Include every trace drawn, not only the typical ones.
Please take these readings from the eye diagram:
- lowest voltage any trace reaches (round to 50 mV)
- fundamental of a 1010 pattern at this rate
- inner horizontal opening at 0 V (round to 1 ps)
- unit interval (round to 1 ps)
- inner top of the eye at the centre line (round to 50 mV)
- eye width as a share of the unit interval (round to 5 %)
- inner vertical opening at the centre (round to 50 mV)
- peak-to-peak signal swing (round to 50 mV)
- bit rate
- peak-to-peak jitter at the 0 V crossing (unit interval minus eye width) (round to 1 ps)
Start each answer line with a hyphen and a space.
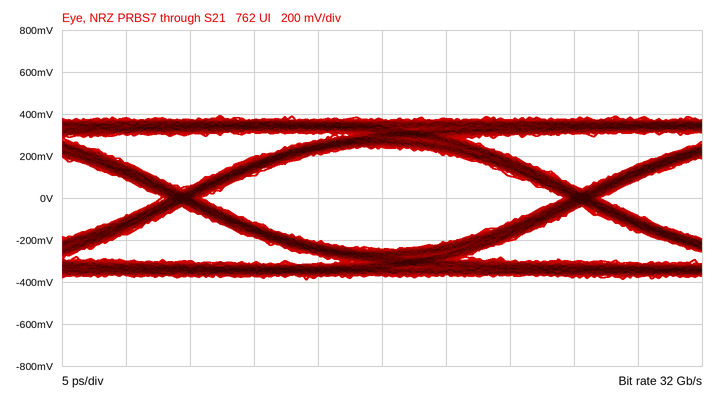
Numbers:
- -400 mV
- 16 GHz
- 28 ps
- 31 ps
- 250 mV
- 90 %
- 500 mV
- 800 mV
- 32 Gb/s
- 3 ps
